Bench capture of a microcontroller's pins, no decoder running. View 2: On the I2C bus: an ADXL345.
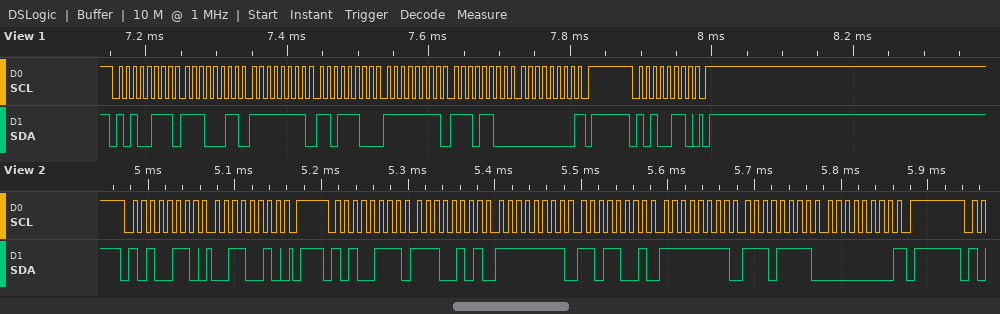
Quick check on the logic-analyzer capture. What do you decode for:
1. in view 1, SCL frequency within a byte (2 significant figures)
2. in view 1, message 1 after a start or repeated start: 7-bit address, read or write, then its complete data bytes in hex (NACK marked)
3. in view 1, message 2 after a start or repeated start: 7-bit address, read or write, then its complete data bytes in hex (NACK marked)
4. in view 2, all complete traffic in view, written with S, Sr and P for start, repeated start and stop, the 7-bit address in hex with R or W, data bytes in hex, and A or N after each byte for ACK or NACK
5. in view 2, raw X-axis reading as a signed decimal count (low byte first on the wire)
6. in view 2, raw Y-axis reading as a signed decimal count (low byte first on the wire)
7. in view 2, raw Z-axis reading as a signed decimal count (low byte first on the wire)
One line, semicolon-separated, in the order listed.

100 kHz; 0x53 read: E3 FF DC FF EC 00 NACK; 0x53 write; S 53W A 32 A P S 53R A E5 A FF A D9 A FF A EF A 00 N P; -27; -39; 239
